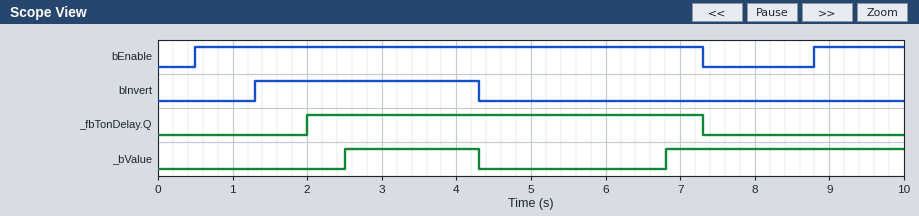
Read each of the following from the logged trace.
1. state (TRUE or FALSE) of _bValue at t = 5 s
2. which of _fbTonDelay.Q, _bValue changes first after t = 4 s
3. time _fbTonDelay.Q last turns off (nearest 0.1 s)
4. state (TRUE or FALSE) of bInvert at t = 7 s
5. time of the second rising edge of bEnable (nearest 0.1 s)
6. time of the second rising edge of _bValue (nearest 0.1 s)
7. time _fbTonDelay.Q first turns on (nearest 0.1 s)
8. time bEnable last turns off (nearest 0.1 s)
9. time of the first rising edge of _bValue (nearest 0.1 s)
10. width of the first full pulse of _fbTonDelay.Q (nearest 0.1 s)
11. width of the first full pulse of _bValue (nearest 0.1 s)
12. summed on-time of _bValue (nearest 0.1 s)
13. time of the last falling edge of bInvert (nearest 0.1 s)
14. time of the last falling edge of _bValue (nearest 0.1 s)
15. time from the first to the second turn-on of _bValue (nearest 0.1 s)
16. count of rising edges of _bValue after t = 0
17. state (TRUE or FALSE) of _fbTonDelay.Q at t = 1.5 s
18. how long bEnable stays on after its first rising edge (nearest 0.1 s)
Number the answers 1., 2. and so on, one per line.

1. FALSE
2. _bValue
3. 7.3 s
4. FALSE
5. 8.8 s
6. 6.8 s
7. 2.0 s
8. 7.3 s
9. 2.5 s
10. 5.3 s
11. 1.8 s
12. 5.0 s
13. 4.3 s
14. 4.3 s
15. 4.3 s
16. 2
17. FALSE
18. 6.8 s
